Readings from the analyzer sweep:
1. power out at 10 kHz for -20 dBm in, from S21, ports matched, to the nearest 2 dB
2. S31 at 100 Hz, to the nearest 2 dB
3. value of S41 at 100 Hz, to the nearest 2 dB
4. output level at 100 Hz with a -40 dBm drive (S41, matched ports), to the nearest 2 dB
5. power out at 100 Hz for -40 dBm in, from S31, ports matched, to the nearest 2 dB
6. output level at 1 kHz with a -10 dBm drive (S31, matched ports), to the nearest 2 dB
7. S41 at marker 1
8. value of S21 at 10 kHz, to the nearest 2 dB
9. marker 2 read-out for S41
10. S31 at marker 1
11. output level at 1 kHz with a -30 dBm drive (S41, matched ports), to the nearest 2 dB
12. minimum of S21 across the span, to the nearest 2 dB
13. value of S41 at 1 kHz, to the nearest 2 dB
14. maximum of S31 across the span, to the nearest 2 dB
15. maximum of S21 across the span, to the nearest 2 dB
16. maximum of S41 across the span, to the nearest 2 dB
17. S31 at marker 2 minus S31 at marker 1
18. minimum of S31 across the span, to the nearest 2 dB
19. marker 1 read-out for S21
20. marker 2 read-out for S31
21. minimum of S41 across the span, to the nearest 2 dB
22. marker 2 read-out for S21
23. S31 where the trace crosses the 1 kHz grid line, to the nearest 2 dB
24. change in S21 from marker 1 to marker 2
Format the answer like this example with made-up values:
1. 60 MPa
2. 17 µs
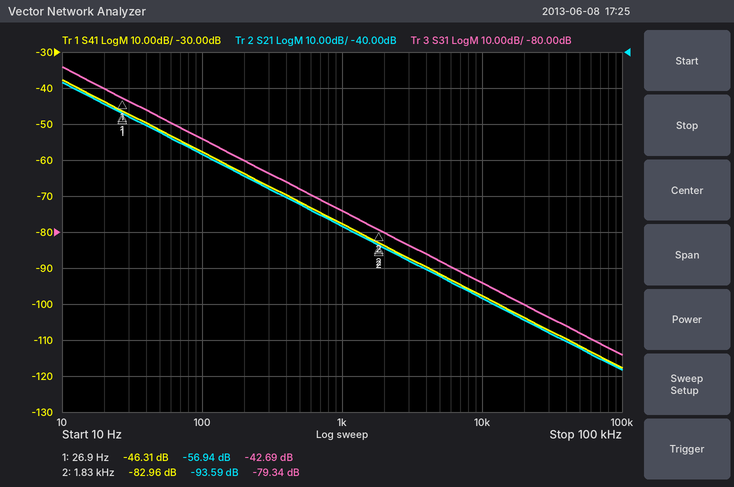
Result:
1. -128 dBm
2. -54 dB
3. -58 dB
4. -98 dBm
5. -94 dBm
6. -84 dBm
7. -46.31 dB
8. -108 dB
9. -82.96 dB
10. -42.69 dB
11. -108 dBm
12. -128 dB
13. -78 dB
14. -34 dB
15. -48 dB
16. -38 dB
17. -36.65 dB
18. -114 dB
19. -56.94 dB
20. -79.34 dB
21. -118 dB
22. -93.59 dB
23. -74 dB
24. -36.65 dB
